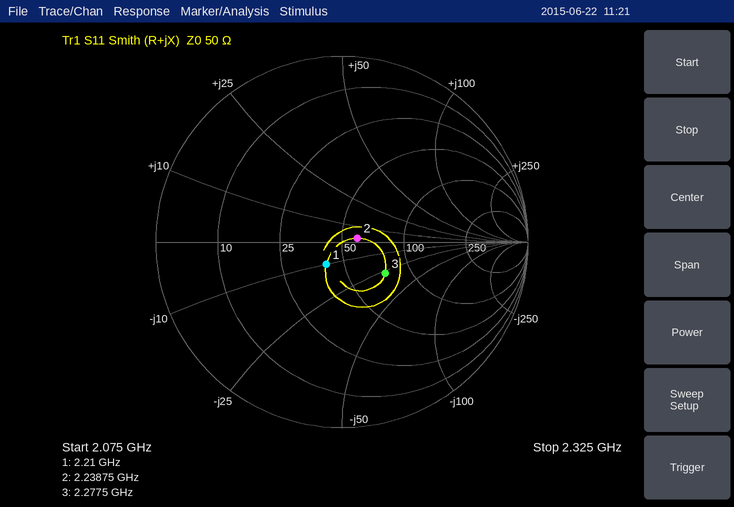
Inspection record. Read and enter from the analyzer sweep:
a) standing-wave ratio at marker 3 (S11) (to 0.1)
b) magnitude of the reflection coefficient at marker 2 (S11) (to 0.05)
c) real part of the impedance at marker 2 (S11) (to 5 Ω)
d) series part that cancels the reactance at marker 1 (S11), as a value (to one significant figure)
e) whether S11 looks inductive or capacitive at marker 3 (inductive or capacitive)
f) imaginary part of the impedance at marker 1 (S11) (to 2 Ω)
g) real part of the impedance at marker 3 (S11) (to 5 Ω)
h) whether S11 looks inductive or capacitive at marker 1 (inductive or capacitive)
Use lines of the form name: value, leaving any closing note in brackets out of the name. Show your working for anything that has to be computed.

standing-wave ratio at marker 3 (S11): 1.8
magnitude of the reflection coefficient at marker 2 (S11): 0.10
real part of the impedance at marker 2 (S11): 60 Ω
series part that cancels the reactance at marker 1 (S11), as a value: L = 10 Ω/(2π × 2.21 GHz) ≈ 720 pH, so 700 pH to one significant figure
whether S11 looks inductive or capacitive at marker 3: capacitive
imaginary part of the impedance at marker 1 (S11): -10 Ω
real part of the impedance at marker 3 (S11): 75 Ω
whether S11 looks inductive or capacitive at marker 1: capacitive
